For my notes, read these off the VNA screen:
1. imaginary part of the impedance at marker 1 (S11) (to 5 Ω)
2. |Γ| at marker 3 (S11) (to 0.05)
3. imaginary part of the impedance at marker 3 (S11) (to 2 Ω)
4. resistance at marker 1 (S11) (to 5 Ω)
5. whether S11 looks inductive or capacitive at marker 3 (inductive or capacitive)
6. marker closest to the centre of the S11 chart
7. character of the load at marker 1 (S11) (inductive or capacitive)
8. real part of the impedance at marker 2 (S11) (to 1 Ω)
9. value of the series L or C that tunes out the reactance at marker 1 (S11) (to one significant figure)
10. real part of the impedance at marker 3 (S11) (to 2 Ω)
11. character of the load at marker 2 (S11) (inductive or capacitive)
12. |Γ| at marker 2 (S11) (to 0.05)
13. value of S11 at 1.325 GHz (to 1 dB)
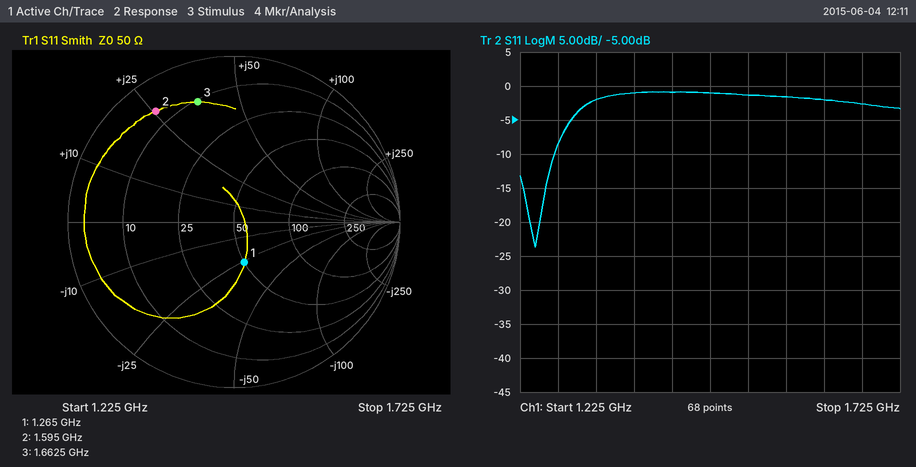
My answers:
-25 Ω
0.75
+36 Ω
50 Ω
inductive
marker 1
capacitive
6 Ω
3 nH
10 Ω
inductive
0.80
-2 dB
